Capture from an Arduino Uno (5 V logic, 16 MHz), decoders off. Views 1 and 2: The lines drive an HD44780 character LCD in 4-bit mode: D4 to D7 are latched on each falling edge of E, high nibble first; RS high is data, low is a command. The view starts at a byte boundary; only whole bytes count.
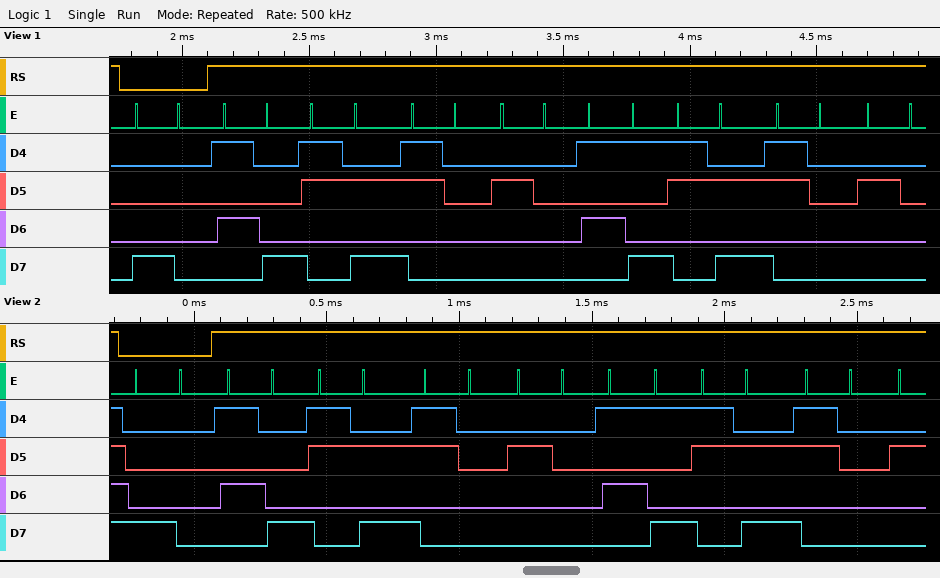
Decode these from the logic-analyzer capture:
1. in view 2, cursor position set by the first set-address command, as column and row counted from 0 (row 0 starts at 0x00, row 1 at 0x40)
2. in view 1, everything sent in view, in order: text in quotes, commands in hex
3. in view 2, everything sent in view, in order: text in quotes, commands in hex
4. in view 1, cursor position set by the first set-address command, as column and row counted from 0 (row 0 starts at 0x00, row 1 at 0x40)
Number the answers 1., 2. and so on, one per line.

1. column 0, row 0
2. 0x80 "X:0 Y:0 "
3. 0x80 "X:0 Y:0"
4. column 0, row 0
